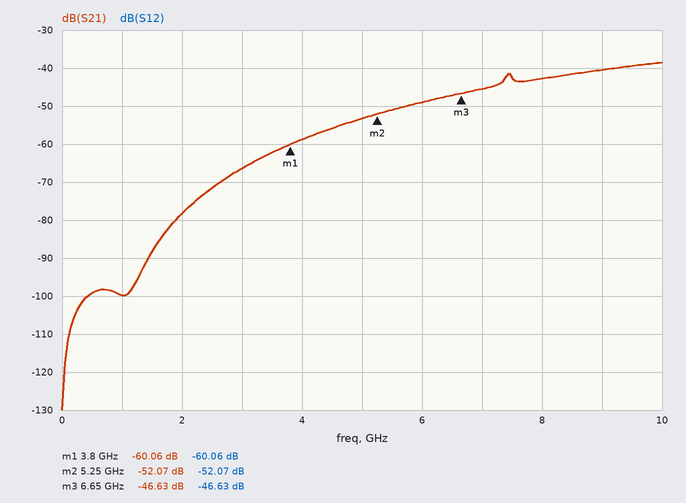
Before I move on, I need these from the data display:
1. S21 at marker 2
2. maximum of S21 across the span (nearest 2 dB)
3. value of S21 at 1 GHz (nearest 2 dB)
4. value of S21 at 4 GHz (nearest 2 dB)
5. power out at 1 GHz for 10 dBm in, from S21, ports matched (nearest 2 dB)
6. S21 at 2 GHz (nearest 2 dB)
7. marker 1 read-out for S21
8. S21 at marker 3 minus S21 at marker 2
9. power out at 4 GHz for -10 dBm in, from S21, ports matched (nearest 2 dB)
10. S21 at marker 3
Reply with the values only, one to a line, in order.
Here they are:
-52.07 dB
-38 dB
-100 dB
-58 dB
-90 dBm
-78 dB
-60.06 dB
5.44 dB
-68 dBm
-46.63 dB
